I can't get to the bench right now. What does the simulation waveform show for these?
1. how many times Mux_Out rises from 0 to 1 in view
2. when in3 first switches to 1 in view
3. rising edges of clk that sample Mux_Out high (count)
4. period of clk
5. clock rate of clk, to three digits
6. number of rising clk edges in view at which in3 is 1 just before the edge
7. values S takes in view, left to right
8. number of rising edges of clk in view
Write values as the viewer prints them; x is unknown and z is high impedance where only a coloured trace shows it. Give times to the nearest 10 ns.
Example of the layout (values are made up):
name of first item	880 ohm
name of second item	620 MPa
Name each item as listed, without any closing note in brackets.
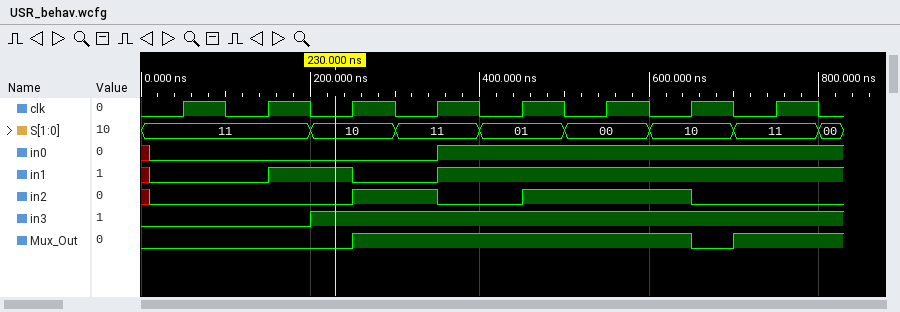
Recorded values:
how many times Mux_Out rises from 0 to 1 in view	2
when in3 first switches to 1 in view	200 ns
rising edges of clk that sample Mux_Out high	5
period of clk	100 ns
clock rate of clk, to three digits	10.0 MHz
number of rising clk edges in view at which in3 is 1 just before the edge	6
values S takes in view, left to right	11, 10, 11, 01, 00, 10, 11, 00
number of rising edges of clk in view	8
